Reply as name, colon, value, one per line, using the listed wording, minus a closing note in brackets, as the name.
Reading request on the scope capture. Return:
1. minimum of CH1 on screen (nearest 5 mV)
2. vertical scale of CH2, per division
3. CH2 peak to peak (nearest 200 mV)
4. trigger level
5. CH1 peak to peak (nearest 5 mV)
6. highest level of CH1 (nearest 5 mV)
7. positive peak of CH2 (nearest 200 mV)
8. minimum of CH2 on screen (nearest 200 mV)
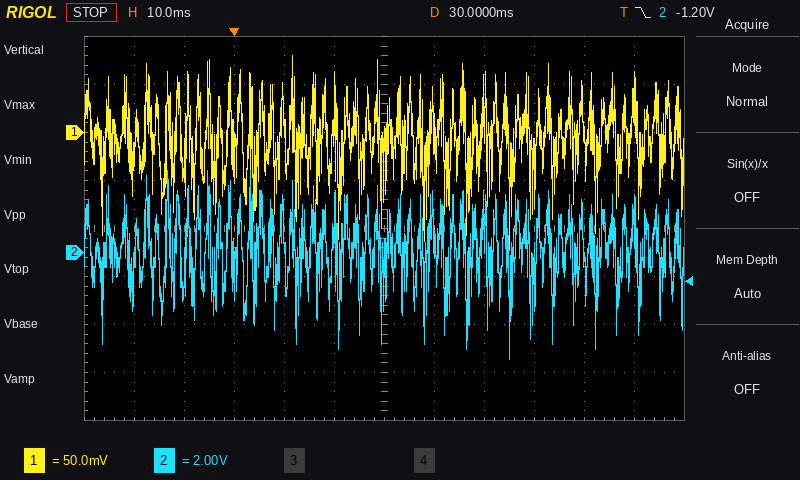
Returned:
minimum of CH1 on screen: -120 mV
vertical scale of CH2, per division: 2 V
CH2 peak to peak: 7.8 V
trigger level: -1.20 V
CH1 peak to peak: 200 mV
highest level of CH1: 80 mV
positive peak of CH2: 3.4 V
minimum of CH2 on screen: -4.4 V
